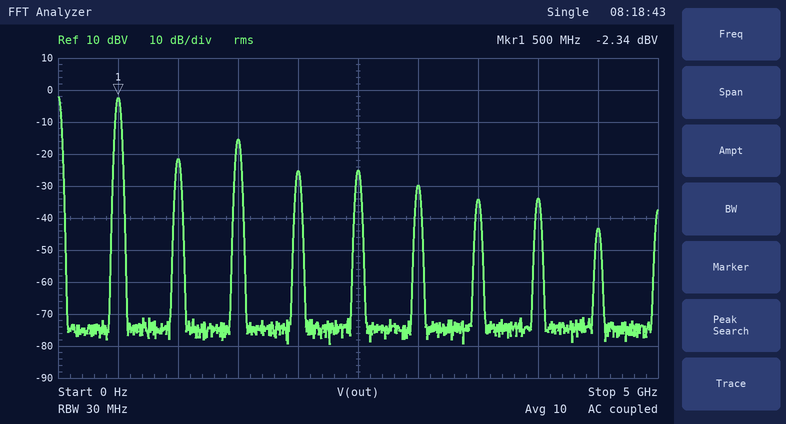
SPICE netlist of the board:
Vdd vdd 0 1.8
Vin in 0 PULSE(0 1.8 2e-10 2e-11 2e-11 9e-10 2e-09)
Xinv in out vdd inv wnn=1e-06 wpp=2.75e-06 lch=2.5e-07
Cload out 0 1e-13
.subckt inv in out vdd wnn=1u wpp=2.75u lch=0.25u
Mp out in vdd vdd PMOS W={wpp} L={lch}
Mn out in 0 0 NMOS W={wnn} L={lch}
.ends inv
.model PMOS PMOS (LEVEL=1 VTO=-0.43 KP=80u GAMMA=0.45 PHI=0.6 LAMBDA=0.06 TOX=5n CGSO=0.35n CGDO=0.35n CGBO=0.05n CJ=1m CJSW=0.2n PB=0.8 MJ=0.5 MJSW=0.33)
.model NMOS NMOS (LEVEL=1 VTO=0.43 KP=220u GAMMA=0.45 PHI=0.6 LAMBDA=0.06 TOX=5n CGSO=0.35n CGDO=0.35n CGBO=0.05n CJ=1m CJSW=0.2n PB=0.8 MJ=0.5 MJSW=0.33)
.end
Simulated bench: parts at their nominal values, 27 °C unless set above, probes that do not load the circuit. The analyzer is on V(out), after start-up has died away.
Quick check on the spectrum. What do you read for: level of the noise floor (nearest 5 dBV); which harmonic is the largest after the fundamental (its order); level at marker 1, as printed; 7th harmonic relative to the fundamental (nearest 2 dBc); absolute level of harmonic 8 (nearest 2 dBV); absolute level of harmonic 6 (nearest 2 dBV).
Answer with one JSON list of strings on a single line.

["-75 dBV", "3", "-2.34 dBV", "-32 dBc", "-34 dBV", "-30 dBV"]
